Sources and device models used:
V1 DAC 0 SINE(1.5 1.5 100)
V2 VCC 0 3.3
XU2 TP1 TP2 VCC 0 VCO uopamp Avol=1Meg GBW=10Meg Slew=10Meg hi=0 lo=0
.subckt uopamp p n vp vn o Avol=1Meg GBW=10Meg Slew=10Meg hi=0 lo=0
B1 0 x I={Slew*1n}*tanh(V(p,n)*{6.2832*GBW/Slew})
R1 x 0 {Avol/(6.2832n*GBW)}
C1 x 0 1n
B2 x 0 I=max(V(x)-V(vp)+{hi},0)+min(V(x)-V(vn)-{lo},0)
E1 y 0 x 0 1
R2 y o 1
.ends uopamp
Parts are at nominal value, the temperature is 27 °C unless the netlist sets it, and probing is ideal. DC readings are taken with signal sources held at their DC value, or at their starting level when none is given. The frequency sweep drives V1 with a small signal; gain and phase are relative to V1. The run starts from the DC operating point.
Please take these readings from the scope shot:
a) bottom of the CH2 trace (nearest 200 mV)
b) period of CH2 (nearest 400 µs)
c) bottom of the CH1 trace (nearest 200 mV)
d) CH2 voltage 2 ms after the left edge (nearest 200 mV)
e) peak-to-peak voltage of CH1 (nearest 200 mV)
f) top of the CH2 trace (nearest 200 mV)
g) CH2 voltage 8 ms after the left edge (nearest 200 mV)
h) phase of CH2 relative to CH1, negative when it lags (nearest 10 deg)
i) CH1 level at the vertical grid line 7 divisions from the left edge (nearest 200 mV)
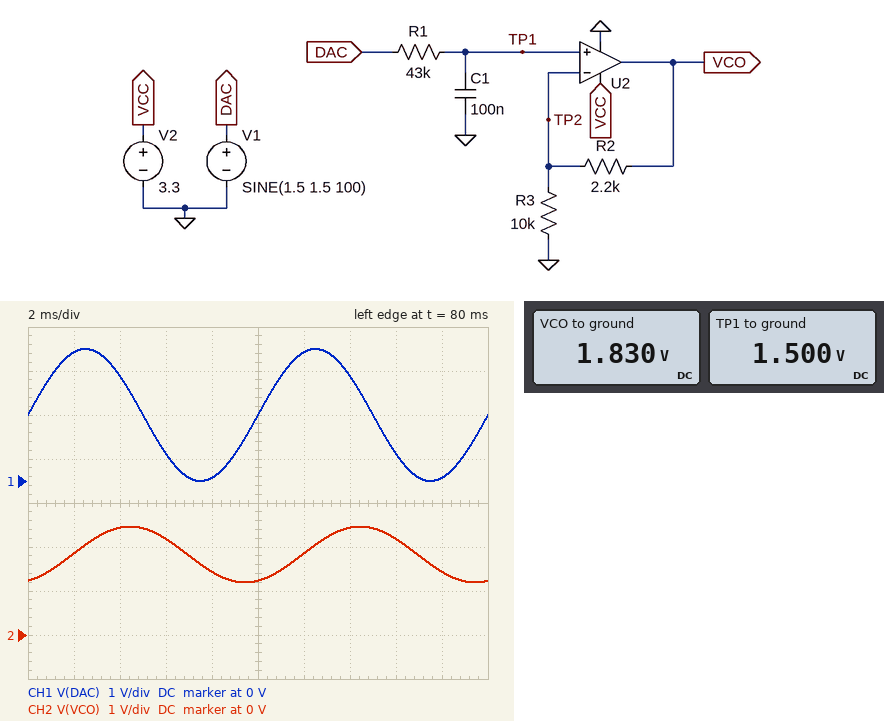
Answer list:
1.2 V
10.0 ms
0 V
1.8 V
3.0 V
2.4 V
1.4 V
-70 deg
2.4 V
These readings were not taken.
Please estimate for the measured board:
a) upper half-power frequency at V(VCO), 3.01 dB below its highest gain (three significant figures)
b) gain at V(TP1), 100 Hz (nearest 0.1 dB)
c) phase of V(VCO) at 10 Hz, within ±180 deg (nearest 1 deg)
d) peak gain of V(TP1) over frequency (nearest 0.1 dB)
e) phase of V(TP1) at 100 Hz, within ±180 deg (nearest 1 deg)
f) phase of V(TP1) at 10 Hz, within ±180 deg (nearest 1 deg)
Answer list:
37.0 Hz
-9.2 dB
-15 deg
0 dB
-70 deg
-15 deg
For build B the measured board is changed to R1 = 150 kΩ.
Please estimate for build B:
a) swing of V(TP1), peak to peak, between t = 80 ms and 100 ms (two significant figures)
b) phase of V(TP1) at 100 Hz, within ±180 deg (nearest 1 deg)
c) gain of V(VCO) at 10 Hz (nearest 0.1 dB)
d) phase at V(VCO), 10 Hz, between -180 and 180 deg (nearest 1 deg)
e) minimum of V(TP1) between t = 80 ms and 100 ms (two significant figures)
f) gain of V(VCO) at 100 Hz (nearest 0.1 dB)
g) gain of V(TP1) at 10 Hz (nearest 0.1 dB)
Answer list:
320 mV
-84 deg
-1.0 dB
-43 deg
1.3 V
-17.8 dB
-2.8 dB
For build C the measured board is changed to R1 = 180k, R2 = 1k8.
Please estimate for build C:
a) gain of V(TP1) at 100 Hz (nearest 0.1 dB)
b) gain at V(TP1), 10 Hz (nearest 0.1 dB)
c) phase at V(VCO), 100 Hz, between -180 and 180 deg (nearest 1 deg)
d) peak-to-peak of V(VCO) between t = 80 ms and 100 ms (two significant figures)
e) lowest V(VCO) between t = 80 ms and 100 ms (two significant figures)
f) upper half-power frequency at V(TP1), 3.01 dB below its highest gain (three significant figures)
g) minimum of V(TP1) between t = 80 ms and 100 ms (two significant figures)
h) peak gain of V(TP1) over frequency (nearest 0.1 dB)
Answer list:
-21.1 dB
-3.6 dB
-85 deg
310 mV
1.6 V
8.84 Hz
1.4 V
0 dB
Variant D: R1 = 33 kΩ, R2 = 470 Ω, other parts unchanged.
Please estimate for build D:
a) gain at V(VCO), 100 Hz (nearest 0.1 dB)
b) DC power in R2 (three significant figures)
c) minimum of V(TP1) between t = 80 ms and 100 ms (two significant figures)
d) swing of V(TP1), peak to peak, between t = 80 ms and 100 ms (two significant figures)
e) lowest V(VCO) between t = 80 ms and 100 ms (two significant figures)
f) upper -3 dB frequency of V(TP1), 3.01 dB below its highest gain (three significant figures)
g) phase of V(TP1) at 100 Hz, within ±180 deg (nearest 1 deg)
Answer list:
-6.8 dB
10.6 µW
850 mV
1.3 V
890 mV
48.2 Hz
-64 deg
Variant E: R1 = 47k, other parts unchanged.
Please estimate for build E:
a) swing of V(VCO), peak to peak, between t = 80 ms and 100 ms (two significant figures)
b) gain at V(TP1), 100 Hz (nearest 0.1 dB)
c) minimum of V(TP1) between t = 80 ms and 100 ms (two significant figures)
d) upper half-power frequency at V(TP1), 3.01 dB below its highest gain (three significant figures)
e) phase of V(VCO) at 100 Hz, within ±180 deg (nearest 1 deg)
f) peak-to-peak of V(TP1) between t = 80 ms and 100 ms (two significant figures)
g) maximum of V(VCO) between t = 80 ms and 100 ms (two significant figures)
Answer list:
1.2 V
-9.9 dB
1.0 V
33.9 Hz
-71 deg
960 mV
2.4 V
